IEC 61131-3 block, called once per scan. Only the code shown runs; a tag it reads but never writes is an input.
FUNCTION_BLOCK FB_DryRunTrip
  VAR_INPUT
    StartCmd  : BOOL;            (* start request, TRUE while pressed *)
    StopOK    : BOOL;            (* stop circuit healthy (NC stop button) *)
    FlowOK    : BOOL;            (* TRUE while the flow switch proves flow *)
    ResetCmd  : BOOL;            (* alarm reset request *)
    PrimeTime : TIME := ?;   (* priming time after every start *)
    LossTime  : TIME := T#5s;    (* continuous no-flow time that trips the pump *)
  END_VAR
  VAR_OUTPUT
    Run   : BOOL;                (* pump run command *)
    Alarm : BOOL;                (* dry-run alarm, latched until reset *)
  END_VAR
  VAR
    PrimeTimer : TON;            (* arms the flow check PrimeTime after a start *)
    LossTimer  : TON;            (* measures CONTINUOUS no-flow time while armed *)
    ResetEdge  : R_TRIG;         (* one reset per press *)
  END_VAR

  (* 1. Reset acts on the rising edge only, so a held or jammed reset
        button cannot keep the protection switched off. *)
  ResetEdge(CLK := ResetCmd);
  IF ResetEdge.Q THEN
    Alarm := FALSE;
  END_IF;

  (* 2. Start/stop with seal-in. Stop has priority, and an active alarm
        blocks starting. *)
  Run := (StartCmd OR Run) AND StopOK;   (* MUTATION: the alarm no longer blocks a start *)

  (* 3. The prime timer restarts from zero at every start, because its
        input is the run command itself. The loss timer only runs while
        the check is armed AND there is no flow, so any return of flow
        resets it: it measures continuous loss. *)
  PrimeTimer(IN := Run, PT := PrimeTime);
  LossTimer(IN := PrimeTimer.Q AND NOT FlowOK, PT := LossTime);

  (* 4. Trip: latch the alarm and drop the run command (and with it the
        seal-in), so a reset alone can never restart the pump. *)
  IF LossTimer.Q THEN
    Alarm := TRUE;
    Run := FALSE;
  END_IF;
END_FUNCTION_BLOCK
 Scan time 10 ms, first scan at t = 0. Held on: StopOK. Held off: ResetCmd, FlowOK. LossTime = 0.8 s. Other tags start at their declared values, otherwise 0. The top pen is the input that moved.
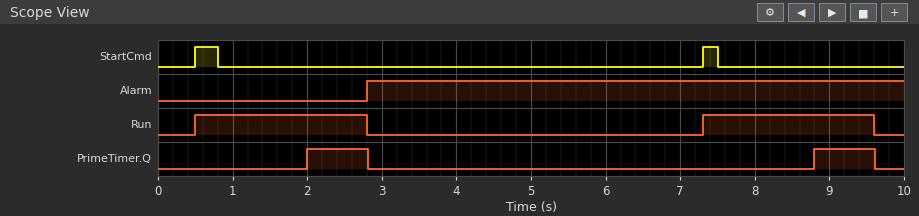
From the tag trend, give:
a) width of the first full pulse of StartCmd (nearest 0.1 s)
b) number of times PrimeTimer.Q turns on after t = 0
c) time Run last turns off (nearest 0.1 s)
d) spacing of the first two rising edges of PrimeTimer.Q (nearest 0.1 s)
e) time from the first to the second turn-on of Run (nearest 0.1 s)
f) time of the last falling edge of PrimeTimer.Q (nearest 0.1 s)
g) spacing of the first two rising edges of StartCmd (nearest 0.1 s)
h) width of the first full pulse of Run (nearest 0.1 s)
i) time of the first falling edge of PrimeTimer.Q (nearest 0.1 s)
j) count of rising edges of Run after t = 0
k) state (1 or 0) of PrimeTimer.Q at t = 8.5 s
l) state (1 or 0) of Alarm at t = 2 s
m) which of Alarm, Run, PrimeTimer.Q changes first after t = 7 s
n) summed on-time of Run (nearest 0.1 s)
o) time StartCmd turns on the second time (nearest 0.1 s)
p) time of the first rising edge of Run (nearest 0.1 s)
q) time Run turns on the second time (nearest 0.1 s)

0.3 s
2
9.6 s
6.8 s
6.8 s
9.6 s
6.8 s
2.3 s
2.8 s
2
0
0
Run
4.6 s
7.3 s
0.5 s
7.3 s
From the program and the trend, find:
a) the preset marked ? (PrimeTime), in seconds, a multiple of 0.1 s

1.5 s
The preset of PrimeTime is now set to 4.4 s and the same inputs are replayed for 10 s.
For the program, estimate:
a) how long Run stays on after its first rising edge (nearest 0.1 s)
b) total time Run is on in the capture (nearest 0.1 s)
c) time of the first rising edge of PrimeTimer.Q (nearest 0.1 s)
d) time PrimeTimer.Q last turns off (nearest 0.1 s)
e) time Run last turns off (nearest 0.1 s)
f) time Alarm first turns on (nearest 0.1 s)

5.2 s
7.9 s
4.9 s
5.7 s
5.7 s
5.7 s
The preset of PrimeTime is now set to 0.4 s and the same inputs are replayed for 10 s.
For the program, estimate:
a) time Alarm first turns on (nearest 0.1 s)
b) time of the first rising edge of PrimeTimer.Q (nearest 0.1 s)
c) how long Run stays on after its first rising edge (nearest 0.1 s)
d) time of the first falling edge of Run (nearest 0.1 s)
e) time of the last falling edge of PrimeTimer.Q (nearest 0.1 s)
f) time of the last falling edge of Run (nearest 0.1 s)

1.7 s
0.9 s
1.2 s
1.7 s
8.5 s
8.5 s
